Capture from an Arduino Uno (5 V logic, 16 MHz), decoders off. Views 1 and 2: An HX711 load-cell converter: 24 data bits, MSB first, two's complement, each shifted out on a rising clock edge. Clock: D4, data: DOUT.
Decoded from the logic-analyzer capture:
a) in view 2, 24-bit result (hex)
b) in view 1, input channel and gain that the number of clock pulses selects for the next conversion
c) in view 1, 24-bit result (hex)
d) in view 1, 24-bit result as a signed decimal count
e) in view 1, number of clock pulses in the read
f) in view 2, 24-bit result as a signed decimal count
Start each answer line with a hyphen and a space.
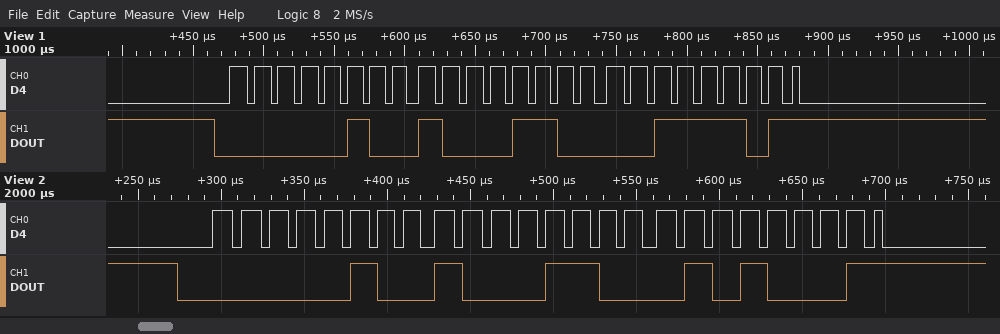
- 0x048C51
- channel A, gain 128
- 0x048C3D
- 298045
- 25
- 298065
